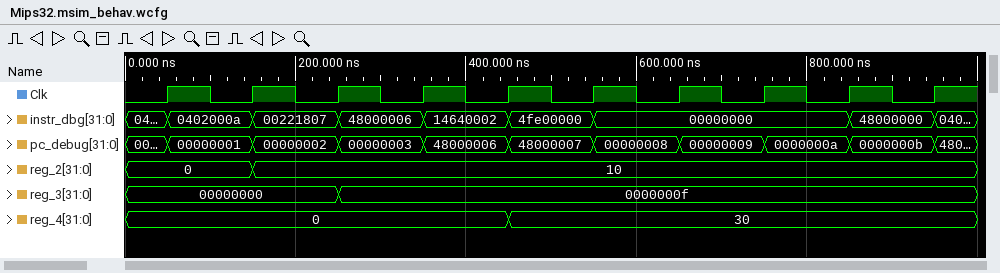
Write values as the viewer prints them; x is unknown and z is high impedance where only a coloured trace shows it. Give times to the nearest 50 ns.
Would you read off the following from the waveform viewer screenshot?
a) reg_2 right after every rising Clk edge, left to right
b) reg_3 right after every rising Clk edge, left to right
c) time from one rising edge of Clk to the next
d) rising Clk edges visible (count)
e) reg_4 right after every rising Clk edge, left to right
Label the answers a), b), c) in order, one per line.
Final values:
a) 0, 10, 10, 10, 10, 10, 10, 10, 10, 10
b) 00000000, 00000000, 0000000f, 0000000f, 0000000f, 0000000f, 0000000f, 0000000f, 0000000f, 0000000f
c) 100 ns
d) 10
e) 0, 0, 0, 0, 30, 30, 30, 30, 30, 30
